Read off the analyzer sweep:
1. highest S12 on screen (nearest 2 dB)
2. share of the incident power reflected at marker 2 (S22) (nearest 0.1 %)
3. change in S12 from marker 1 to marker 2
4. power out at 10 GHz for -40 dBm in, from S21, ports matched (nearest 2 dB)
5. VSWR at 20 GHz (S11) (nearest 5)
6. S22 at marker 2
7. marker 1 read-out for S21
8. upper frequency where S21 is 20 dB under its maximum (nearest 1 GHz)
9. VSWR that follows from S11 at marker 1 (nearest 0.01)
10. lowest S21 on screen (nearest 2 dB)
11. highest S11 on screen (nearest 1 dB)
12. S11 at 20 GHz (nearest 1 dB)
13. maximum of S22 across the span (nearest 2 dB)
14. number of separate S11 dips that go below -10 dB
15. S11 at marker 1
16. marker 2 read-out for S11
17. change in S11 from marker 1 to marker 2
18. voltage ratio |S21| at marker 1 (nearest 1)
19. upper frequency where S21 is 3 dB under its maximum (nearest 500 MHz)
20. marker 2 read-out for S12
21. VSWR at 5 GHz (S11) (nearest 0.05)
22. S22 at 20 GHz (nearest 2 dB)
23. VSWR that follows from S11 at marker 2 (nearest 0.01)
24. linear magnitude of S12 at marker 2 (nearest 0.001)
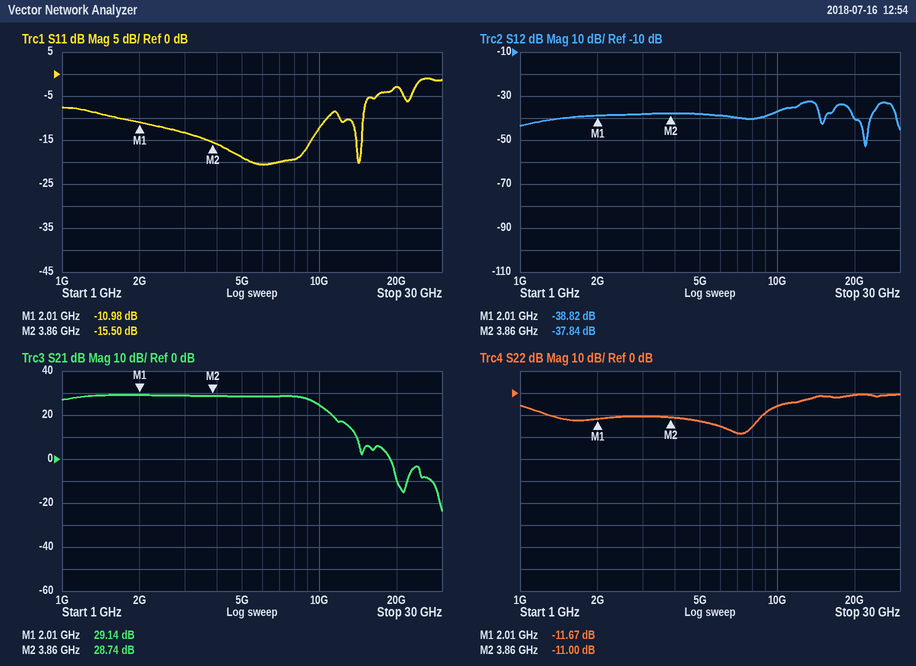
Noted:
-32 dB
7.9 %
0.98 dB
-16 dBm
5
-11.00 dB
29.14 dB
14 GHz
1.79
-24 dB
-1 dB
-3 dB
0 dB
2
-10.98 dB
-15.50 dB
-4.52 dB
29
9.5 GHz
-37.84 dB
1.25
0 dB
1.40
0.013
